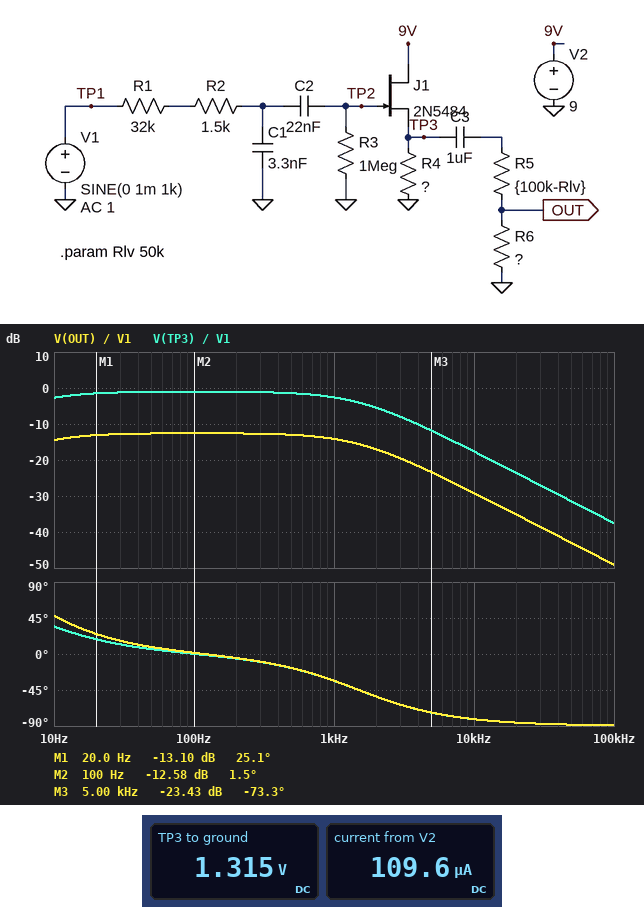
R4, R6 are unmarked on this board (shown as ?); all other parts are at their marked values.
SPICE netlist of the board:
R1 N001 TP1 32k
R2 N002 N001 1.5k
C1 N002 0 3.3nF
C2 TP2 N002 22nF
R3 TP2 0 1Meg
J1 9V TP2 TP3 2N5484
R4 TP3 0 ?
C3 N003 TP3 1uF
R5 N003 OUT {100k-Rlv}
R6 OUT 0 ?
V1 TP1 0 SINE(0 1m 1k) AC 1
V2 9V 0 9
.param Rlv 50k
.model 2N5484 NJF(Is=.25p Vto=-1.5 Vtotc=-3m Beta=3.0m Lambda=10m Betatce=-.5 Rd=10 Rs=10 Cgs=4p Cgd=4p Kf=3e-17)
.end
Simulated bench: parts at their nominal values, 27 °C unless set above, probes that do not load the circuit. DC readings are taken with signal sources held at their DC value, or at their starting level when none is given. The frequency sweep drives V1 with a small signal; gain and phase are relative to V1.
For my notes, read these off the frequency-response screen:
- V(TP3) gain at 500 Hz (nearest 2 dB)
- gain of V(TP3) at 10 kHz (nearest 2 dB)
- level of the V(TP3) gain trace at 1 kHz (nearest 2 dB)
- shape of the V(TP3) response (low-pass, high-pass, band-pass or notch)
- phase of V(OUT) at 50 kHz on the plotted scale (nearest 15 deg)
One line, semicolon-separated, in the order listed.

-2 dB; -18 dB; -2 dB; low-pass; -90 deg
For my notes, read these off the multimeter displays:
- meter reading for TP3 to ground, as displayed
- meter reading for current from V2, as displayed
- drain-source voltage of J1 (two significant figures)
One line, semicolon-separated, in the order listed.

1.315 V; 109.6 µA; 7.7 V
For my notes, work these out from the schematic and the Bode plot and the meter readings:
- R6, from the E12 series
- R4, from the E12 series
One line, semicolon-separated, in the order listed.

18 kΩ; 12 kΩ
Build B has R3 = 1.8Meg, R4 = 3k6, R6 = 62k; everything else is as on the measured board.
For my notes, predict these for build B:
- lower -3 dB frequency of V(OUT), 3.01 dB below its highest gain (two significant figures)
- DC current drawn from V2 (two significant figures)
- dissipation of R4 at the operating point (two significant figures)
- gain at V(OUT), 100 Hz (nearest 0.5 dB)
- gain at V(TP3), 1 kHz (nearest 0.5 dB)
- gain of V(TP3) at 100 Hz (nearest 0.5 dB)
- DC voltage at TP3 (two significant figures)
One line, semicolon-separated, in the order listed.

4.4 Hz; 330 µA; 390 µW; -6.5 dB; -3.0 dB; -1.5 dB; 1.2 V
